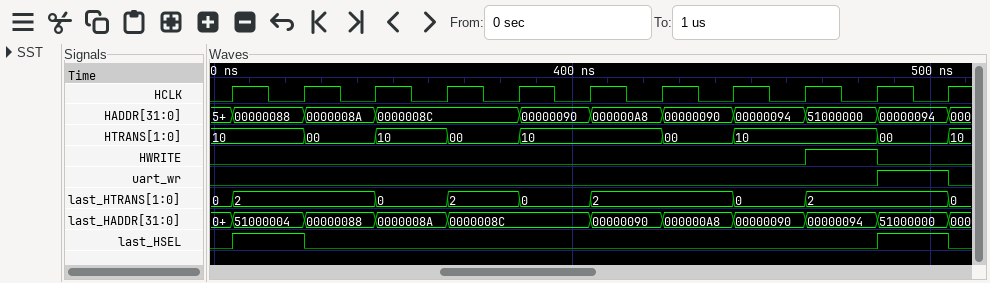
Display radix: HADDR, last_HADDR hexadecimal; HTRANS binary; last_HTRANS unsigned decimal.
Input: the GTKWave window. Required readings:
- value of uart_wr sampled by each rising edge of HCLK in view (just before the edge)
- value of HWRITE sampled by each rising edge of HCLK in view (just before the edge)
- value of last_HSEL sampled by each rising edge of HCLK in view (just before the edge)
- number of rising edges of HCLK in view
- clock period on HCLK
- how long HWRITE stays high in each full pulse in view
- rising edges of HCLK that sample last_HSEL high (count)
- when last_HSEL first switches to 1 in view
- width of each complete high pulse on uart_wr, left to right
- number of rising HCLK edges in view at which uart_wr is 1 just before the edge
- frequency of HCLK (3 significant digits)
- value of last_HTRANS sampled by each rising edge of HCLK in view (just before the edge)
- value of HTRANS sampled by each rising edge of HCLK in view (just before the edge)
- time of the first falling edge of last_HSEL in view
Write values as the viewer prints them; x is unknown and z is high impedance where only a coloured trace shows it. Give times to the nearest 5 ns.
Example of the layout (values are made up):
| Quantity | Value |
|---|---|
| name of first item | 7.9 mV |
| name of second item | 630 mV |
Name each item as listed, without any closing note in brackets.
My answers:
| Quantity | Value |
|---|---|
| value of uart_wr sampled by each rising edge of HCLK in view | 0 0 0 0 0 0 0 0 0 0 1 |
| value of HWRITE sampled by each rising edge of HCLK in view | 0 0 0 0 0 0 0 0 0 1 0 |
| value of last_HSEL sampled by each rising edge of HCLK in view | 0 1 0 0 0 0 0 0 0 0 1 |
| number of rising edges of HCLK in view | 11 |
| clock period on HCLK | 20 ns |
| how long HWRITE stays high in each full pulse in view | 20 ns |
| rising edges of HCLK that sample last_HSEL high | 2 |
| when last_HSEL first switches to 1 in view | 305 ns |
| width of each complete high pulse on uart_wr, left to right | 20 ns |
| number of rising HCLK edges in view at which uart_wr is 1 just before the edge | 1 |
| frequency of HCLK | 50.0 MHz |
| value of last_HTRANS sampled by each rising edge of HCLK in view | 0, 2, 2, 0, 2, 0, 2, 2, 0, 2, 2 |
| value of HTRANS sampled by each rising edge of HCLK in view | 10, 10, 00, 10, 00, 10, 10, 00, 10, 10, 00 |
| time of the first falling edge of last_HSEL in view | 325 ns |
